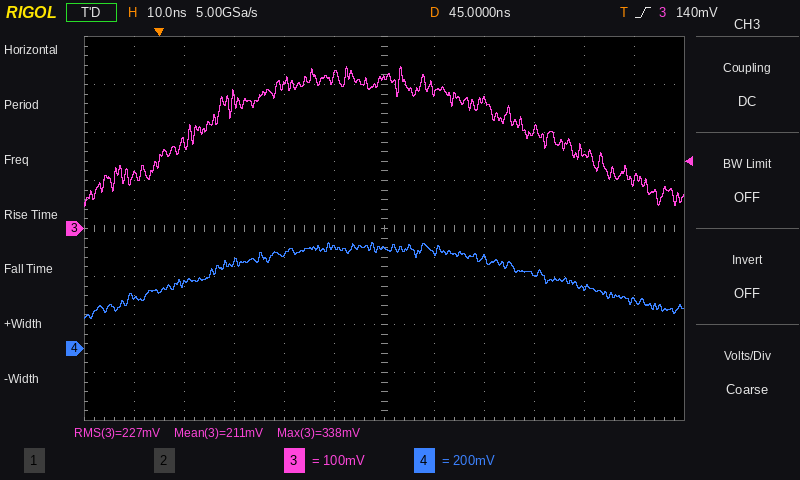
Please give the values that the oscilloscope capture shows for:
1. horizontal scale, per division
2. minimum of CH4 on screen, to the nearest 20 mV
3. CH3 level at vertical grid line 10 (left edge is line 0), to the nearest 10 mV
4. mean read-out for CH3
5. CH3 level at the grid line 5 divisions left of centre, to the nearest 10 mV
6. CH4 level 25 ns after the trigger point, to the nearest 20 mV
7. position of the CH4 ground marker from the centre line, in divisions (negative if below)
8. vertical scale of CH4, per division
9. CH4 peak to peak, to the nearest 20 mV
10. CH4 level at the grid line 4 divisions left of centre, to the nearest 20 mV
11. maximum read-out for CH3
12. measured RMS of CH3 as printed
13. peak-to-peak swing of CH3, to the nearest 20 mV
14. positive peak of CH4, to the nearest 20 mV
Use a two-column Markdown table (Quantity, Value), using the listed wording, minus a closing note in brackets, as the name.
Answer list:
| Quantity | Value |
|---|---|
| horizontal scale, per division | 10 ns |
| minimum of CH4 on screen, to the nearest 20 mV | 120 mV |
| CH3 level at vertical grid line 10 (left edge is line 0), to the nearest 10 mV | 160 mV |
| mean read-out for CH3 | 211 mV |
| CH3 level at the grid line 5 divisions left of centre, to the nearest 10 mV | 110 mV |
| CH4 level 25 ns after the trigger point, to the nearest 20 mV | 400 mV |
| position of the CH4 ground marker from the centre line, in divisions | -2.5 div |
| vertical scale of CH4, per division | 200 mV |
| CH4 peak to peak, to the nearest 20 mV | 320 mV |
| CH4 level at the grid line 4 divisions left of centre, to the nearest 20 mV | 260 mV |
| maximum read-out for CH3 | 338 mV |
| measured RMS of CH3 as printed | 227 mV |
| peak-to-peak swing of CH3, to the nearest 20 mV | 300 mV |
| positive peak of CH4, to the nearest 20 mV | 440 mV |
